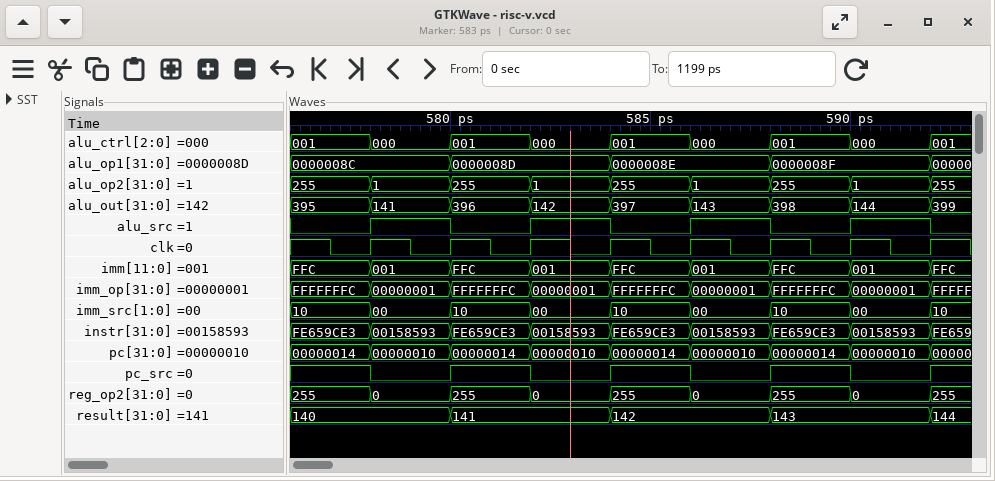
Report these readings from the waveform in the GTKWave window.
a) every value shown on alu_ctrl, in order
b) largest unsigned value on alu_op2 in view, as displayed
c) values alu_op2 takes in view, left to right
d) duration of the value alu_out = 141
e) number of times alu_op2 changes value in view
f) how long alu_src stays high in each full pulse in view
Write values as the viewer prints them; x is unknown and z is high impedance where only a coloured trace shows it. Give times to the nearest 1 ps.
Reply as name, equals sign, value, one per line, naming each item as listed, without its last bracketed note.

every value shown on alu_ctrl, in order = 001, 000, 001, 000, 001, 000, 001, 000, 001
largest unsigned value on alu_op2 in view, as displayed = 255
values alu_op2 takes in view, left to right = 255, 1, 255, 1, 255, 1, 255, 1, 255
duration of the value alu_out = 141 = 2 ps
number of times alu_op2 changes value in view = 8
how long alu_src stays high in each full pulse in view = 2 ps, 2 ps, 2 ps, 2 ps
